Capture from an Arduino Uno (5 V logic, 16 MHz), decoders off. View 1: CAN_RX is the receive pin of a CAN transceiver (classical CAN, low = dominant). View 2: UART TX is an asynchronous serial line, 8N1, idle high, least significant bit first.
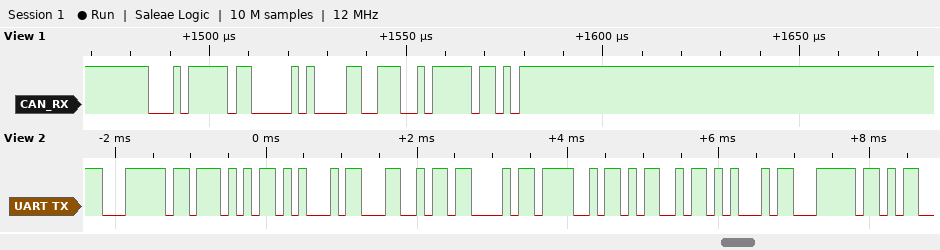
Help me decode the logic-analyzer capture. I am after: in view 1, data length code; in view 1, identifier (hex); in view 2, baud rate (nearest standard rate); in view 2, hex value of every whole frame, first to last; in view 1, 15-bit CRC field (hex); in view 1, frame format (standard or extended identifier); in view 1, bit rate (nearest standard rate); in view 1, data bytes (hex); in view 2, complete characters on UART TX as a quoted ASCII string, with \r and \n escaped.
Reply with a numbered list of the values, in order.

1. 1
2. 0x17F
3. 9600 baud
4. 7C 57 45 4C 43 4F 4D 45 7C
5. 0x72FE
6. standard
7. 500 kbit/s
8. 0C
9. "|WELCOME|"
